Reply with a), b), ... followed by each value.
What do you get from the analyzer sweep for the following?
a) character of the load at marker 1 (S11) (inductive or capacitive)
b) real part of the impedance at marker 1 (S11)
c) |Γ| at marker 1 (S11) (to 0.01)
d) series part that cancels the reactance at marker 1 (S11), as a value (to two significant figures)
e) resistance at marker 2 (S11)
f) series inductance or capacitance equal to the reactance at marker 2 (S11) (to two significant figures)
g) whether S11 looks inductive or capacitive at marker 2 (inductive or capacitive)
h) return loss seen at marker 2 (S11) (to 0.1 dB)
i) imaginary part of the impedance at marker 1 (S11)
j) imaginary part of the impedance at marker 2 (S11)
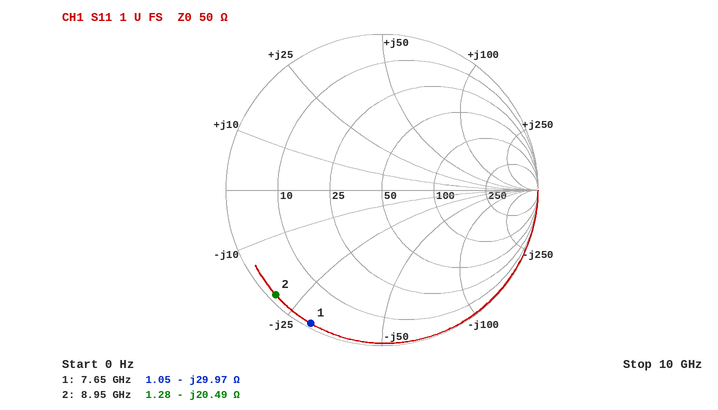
a) capacitive
b) 1.05 Ω
c) 0.97
d) 620 pH
e) 1.28 Ω
f) 870 fF
g) capacitive
h) 0.4 dB
i) -29.97 Ω
j) -20.49 Ω
